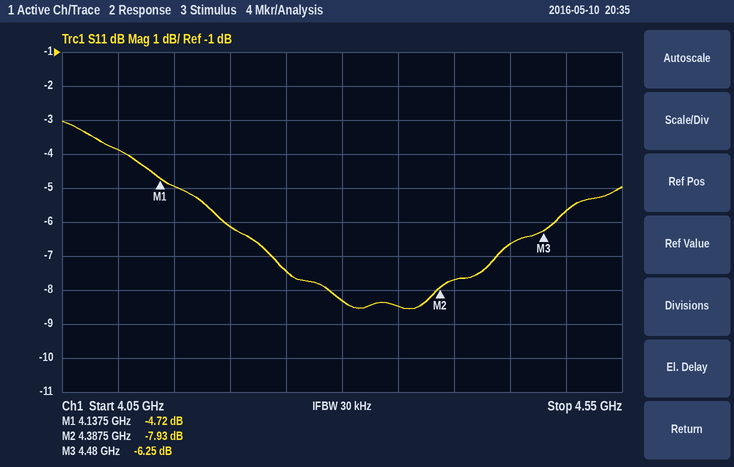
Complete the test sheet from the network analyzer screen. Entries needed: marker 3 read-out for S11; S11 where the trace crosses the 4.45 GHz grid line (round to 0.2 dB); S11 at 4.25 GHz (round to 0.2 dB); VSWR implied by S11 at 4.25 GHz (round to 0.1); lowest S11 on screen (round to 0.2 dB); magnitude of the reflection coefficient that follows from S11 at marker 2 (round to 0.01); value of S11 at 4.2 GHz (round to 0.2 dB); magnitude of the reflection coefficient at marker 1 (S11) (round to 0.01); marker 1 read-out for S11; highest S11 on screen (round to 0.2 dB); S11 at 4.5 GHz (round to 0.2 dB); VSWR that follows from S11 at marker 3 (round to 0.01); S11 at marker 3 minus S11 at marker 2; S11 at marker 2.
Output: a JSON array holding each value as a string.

["-6.25 dB", "-6.6 dB", "-7.4 dB", "2.5", "-8.6 dB", "0.40", "-6.2 dB", "0.58", "-4.72 dB", "-3.0 dB", "-5.6 dB", "2.90", "1.68 dB", "-7.93 dB"]
